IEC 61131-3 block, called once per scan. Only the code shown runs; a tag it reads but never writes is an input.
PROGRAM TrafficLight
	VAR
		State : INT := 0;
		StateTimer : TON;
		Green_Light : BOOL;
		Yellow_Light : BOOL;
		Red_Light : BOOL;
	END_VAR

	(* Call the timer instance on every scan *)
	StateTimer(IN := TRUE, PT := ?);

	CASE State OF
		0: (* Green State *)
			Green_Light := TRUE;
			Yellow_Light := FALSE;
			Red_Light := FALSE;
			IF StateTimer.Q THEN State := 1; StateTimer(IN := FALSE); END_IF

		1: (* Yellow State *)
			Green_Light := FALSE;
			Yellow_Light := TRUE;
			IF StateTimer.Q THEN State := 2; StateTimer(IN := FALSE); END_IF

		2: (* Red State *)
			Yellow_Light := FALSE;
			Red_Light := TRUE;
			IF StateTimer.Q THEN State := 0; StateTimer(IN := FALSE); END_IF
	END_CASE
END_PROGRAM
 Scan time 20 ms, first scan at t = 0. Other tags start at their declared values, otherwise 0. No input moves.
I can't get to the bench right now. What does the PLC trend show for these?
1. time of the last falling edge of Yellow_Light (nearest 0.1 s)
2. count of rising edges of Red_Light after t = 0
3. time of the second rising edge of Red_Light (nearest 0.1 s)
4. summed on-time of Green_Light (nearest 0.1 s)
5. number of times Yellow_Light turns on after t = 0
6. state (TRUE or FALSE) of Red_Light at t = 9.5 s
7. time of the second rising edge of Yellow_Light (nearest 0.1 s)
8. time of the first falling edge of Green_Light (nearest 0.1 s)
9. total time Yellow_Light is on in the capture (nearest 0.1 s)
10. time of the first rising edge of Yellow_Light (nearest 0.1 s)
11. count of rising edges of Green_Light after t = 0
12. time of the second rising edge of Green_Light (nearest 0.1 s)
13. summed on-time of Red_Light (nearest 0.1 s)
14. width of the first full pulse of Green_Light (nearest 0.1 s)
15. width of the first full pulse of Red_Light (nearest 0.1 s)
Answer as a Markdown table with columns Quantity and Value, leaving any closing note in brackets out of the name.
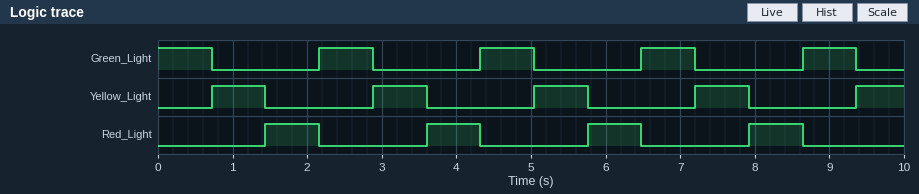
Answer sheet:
| Quantity | Value |
|---|---|
| time of the last falling edge of Yellow_Light | 7.9 s |
| count of rising edges of Red_Light after t = 0 | 4 |
| time of the second rising edge of Red_Light | 3.6 s |
| summed on-time of Green_Light | 3.6 s |
| number of times Yellow_Light turns on after t = 0 | 5 |
| state (TRUE or FALSE) of Red_Light at t = 9.5 s | FALSE |
| time of the second rising edge of Yellow_Light | 2.9 s |
| time of the first falling edge of Green_Light | 0.7 s |
| total time Yellow_Light is on in the capture | 3.5 s |
| time of the first rising edge of Yellow_Light | 0.7 s |
| count of rising edges of Green_Light after t = 0 | 4 |
| time of the second rising edge of Green_Light | 4.3 s |
| summed on-time of Red_Light | 2.9 s |
| width of the first full pulse of Green_Light | 0.7 s |
| width of the first full pulse of Red_Light | 0.7 s |
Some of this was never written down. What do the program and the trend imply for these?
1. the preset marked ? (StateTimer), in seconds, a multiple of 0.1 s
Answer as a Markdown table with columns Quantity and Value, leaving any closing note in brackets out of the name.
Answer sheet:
| Quantity | Value |
|---|---|
| the preset marked ? (StateTimer), in seconds, a multiple of 0.1 s | 0.7 s |
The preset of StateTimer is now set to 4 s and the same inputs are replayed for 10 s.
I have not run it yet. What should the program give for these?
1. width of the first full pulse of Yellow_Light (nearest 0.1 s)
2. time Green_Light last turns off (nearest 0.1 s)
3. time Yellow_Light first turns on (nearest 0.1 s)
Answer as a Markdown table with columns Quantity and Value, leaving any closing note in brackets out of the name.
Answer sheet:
| Quantity | Value |
|---|---|
| width of the first full pulse of Yellow_Light | 4.0 s |
| time Green_Light last turns off | 4.0 s |
| time Yellow_Light first turns on | 4.0 s |
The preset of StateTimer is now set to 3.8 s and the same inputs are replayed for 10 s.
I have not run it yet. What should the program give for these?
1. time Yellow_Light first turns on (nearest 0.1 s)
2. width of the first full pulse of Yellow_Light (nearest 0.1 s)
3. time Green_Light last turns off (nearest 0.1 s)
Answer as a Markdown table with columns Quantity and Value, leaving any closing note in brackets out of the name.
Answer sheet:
| Quantity | Value |
|---|---|
| time Yellow_Light first turns on | 3.8 s |
| width of the first full pulse of Yellow_Light | 3.8 s |
| time Green_Light last turns off | 3.8 s |
